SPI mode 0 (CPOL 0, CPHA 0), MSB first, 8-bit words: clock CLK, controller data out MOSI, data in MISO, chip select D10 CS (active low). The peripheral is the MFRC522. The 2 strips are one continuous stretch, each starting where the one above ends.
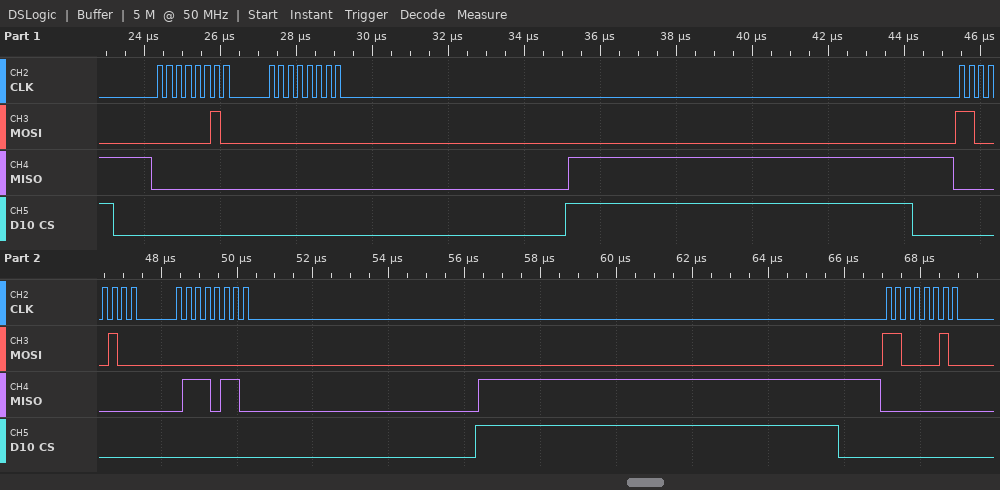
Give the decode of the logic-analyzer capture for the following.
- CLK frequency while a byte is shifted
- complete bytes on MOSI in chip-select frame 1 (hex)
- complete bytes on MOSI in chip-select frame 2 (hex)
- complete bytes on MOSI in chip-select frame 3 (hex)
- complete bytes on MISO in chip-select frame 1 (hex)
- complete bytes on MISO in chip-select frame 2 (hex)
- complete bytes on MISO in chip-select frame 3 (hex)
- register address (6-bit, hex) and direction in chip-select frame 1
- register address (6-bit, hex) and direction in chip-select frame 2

4 MHz
02 00
C4 00
C2
00 00
00 76
00
0x01 write
0x22 read
